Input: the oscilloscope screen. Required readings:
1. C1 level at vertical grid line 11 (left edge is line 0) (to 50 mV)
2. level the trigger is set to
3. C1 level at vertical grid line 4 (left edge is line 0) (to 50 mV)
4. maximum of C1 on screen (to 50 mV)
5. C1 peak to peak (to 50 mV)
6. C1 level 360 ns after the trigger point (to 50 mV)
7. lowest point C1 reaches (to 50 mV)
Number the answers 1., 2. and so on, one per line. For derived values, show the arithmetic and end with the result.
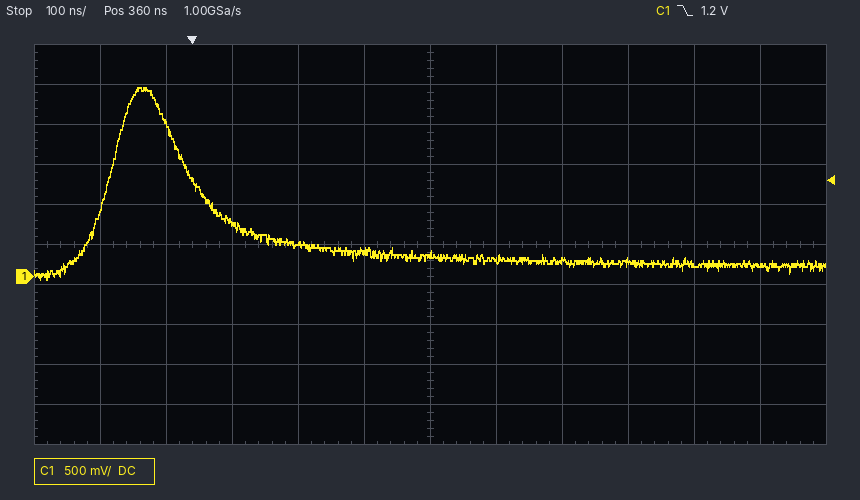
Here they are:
1. 150 mV
2. 1.2 V
3. 400 mV
4. 2.35 V
5. 2.35 V − (-50 mV) = 2.40 V
6. 300 mV
7. -50 mV
